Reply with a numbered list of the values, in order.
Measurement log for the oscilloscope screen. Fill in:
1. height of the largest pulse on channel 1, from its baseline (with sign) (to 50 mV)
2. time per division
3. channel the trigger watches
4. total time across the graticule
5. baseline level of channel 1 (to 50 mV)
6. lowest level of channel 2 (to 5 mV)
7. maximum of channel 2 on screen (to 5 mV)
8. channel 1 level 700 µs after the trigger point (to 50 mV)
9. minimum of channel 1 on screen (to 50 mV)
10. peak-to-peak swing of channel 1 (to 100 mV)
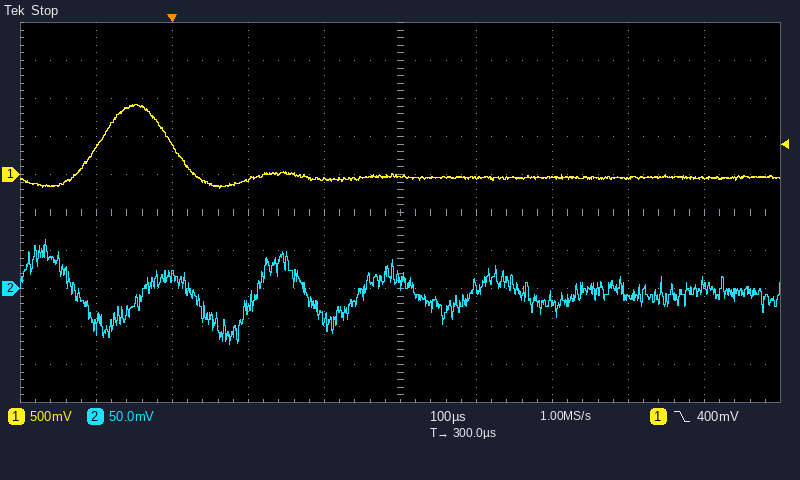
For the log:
1. +950 mV
2. 100 µs
3. channel 1
4. 1 ms
5. -50 mV
6. -75 mV
7. 65 mV
8. -50 mV
9. -200 mV
10. 1.10 V
